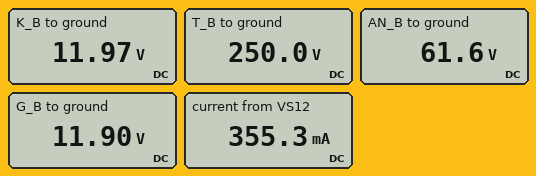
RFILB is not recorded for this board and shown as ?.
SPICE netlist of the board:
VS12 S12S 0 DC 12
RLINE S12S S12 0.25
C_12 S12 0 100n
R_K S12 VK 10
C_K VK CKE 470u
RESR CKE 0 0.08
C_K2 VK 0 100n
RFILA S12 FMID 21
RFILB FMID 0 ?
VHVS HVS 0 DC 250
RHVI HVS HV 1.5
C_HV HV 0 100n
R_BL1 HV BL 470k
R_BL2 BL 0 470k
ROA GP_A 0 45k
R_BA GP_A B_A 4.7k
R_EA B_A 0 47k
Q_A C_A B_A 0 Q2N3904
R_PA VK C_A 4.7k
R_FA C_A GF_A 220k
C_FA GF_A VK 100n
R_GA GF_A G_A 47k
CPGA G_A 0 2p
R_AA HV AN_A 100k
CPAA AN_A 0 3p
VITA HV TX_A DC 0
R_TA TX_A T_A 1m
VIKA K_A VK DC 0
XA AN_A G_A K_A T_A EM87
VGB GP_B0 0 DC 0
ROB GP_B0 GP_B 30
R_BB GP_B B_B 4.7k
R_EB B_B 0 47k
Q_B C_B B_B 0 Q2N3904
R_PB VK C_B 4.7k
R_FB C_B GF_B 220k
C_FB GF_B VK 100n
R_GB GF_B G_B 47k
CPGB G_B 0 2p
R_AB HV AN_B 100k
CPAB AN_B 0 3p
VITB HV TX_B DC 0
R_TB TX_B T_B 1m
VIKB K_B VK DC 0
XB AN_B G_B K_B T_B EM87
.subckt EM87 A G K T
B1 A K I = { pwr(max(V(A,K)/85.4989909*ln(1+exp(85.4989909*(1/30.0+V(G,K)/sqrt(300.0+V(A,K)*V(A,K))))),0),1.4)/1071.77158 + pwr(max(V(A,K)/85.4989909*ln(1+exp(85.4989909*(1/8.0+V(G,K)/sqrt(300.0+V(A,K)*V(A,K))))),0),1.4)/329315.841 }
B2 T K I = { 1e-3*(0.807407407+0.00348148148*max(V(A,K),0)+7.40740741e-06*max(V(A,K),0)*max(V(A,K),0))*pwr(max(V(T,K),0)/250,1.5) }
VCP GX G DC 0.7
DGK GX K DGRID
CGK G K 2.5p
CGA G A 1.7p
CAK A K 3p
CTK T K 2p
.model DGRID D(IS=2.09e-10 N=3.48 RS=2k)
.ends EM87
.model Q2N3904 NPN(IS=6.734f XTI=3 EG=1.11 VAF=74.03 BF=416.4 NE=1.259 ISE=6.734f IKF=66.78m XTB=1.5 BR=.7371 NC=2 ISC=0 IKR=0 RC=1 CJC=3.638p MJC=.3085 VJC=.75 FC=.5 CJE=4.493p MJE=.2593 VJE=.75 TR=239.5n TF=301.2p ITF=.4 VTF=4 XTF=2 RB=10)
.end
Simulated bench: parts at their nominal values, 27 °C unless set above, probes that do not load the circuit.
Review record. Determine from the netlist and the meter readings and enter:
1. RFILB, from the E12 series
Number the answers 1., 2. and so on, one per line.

1. 12 Ω
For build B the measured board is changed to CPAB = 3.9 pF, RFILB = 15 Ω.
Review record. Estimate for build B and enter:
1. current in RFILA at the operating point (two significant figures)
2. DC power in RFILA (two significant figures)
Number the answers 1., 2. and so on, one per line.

1. 330 mA
2. 2.3 W
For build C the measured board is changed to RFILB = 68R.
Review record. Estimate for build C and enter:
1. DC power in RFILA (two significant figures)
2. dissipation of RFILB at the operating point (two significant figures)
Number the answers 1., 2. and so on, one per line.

1. 380 mW
2. 1.2 W
